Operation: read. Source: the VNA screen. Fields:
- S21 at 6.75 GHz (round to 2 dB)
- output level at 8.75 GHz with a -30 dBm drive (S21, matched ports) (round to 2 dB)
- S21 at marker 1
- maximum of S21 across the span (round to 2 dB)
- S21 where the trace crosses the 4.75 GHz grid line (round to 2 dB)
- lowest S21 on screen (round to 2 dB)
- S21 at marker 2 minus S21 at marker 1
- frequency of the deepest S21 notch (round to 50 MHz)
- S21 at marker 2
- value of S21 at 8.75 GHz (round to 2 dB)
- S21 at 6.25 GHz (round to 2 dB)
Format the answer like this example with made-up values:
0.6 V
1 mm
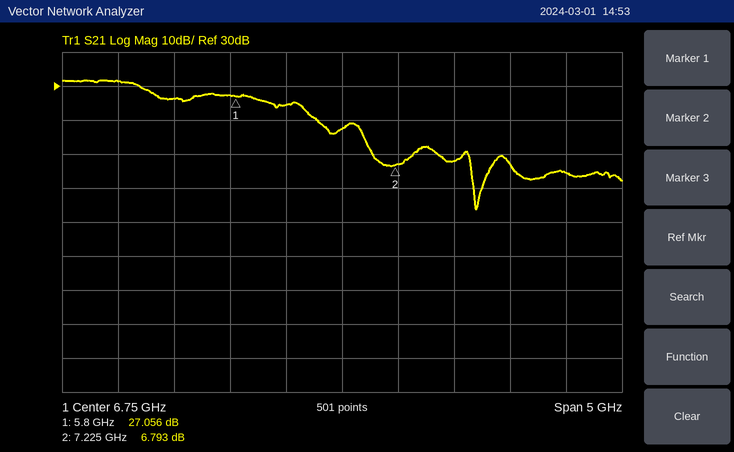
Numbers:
18 dB
-26 dBm
27.056 dB
32 dB
32 dB
-6 dB
-20.263 dB
7.95 GHz
6.793 dB
4 dB
24 dB
